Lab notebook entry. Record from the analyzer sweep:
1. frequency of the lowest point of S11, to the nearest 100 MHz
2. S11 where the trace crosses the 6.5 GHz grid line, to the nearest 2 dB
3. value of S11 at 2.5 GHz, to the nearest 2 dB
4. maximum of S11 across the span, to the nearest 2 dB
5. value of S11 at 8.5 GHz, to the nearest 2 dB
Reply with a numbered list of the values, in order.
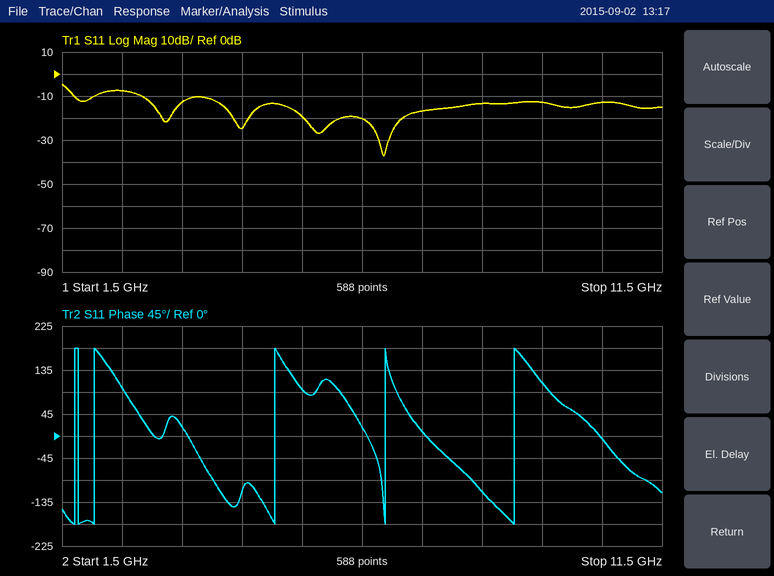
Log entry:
1. 6.9 GHz
2. -20 dB
3. -8 dB
4. -4 dB
5. -14 dB
